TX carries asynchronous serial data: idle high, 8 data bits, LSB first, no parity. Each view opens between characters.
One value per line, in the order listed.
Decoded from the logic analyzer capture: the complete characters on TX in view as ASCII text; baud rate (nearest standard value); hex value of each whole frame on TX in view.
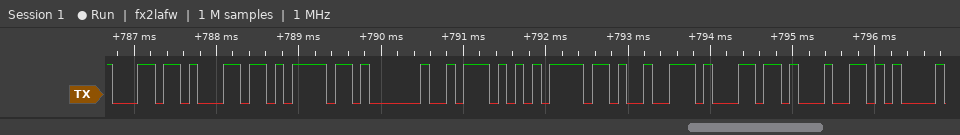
"llo World"
9600 baud
6C, 6C, 6F, 20, 57, 6F, 72, 6C, 64
